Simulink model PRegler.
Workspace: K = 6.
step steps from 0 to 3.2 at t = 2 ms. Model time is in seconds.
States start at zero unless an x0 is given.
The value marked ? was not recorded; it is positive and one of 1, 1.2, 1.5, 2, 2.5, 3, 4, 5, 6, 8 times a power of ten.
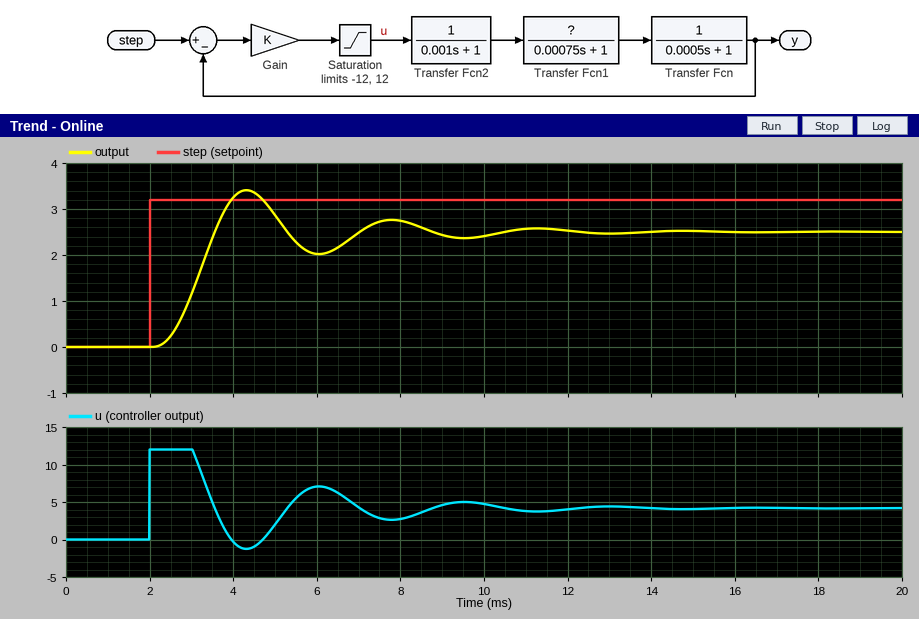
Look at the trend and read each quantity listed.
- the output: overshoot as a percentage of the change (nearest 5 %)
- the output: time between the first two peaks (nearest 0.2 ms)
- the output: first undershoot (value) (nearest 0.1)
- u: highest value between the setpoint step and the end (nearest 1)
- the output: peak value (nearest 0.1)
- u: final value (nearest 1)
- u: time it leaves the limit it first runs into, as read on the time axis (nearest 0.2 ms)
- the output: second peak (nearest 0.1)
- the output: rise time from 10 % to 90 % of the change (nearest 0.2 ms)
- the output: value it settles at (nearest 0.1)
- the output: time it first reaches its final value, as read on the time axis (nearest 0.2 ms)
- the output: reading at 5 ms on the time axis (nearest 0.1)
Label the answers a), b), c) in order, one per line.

a) 35 %
b) 3.4 ms
c) 2.0
d) 12
e) 3.4
f) 4
g) 3.0 ms
h) 2.8
i) 1.0 ms
j) 2.5
k) 3.6 ms
l) 2.9
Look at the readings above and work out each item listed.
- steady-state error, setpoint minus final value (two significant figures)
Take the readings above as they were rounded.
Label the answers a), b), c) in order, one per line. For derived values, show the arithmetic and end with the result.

a) 3.2 - 2.5 = 0.70
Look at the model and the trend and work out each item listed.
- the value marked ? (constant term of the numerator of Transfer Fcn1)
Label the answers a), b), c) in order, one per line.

a) 0.6
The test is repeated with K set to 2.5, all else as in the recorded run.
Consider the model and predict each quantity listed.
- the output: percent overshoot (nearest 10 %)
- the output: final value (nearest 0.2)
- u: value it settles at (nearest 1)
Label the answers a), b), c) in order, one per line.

a) 20 %
b) 2.0
c) 3
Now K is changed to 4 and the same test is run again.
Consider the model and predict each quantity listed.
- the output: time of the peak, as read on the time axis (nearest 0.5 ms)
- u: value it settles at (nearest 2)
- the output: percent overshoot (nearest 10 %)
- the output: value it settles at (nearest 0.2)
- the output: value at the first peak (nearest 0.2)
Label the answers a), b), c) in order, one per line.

a) 4.5 ms
b) 4
c) 30 %
d) 2.2
e) 3.0
